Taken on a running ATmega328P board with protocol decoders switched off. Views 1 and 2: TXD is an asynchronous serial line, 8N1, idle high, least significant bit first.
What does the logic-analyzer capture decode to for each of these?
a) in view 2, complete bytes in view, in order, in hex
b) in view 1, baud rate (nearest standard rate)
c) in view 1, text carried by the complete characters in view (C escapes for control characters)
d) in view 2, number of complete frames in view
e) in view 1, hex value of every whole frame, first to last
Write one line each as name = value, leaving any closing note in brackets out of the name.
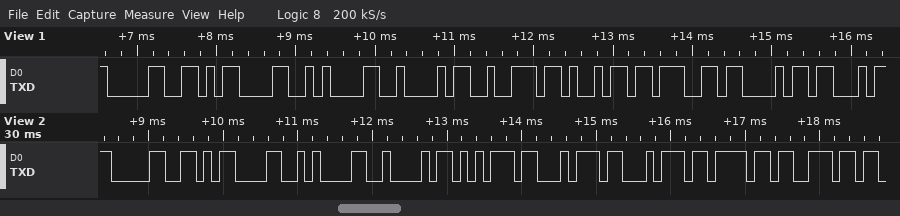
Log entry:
in view 2, complete bytes in view, in order, in hex = 0x30 0x0D 0x0A 0x42 0x75 0x74 0x74 0x6F 0x6E
in view 1, baud rate = 9600 baud
in view 1, text carried by the complete characters in view = "0\r\nBrigh"
in view 2, number of complete frames in view = 9
in view 1, hex value of every whole frame, first to last = 0x30 0x0D 0x0A 0x42 0x72 0x69 0x67 0x68
